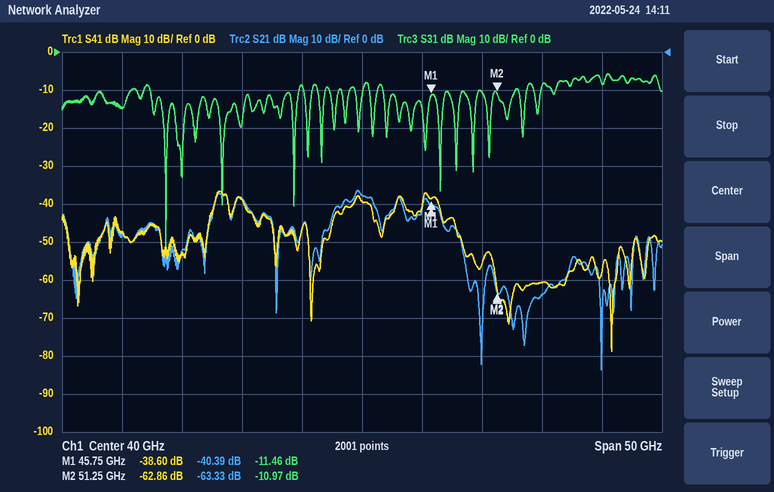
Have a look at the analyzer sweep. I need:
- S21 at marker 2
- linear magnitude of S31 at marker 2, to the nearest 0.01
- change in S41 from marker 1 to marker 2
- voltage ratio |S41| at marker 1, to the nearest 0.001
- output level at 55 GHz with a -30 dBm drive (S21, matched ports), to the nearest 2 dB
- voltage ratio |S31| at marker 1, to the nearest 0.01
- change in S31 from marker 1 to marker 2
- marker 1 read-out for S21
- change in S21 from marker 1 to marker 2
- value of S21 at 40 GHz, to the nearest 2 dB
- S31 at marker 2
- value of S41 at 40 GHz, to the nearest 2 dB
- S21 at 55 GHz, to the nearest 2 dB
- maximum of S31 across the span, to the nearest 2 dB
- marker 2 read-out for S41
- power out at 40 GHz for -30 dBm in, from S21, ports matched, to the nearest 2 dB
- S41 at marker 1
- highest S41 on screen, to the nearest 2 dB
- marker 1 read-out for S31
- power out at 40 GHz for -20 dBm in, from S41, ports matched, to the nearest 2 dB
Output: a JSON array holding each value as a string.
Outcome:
["-63.33 dB", "0.28", "-24.26 dB", "0.012", "-94 dBm", "0.27", "0.49 dB", "-40.39 dB", "-22.94 dB", "-38 dB", "-10.97 dB", "-40 dB", "-64 dB", "-6 dB", "-62.86 dB", "-68 dBm", "-38.60 dB", "-36 dB", "-11.46 dB", "-60 dBm"]
